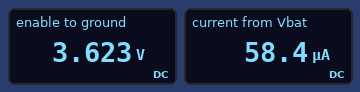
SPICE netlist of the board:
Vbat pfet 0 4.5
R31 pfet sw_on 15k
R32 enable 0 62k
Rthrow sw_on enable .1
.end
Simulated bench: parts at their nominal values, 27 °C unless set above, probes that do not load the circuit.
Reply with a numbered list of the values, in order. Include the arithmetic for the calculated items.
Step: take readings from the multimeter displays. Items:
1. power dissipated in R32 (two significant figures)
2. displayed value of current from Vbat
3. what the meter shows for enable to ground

1. (3.623 V)^2 / 62 kΩ = 210 µW
2. 58.4 µA
3. 3.623 V
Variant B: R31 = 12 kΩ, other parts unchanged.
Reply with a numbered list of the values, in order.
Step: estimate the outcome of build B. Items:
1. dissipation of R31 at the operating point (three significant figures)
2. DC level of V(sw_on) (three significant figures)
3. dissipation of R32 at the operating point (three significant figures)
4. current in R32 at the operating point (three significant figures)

1. 44.4 µW
2. 3.77 V
3. 229 µW
4. 60.8 µA
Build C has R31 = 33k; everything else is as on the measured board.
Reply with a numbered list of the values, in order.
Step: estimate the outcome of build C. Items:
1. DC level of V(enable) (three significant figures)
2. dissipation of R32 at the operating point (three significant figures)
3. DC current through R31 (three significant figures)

1. 2.94 V
2. 139 µW
3. 47.4 µA
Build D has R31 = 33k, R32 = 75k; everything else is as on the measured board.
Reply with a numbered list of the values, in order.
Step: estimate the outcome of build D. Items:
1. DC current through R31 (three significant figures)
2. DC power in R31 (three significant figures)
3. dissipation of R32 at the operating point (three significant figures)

1. 41.7 µA
2. 57.3 µW
3. 130 µW
